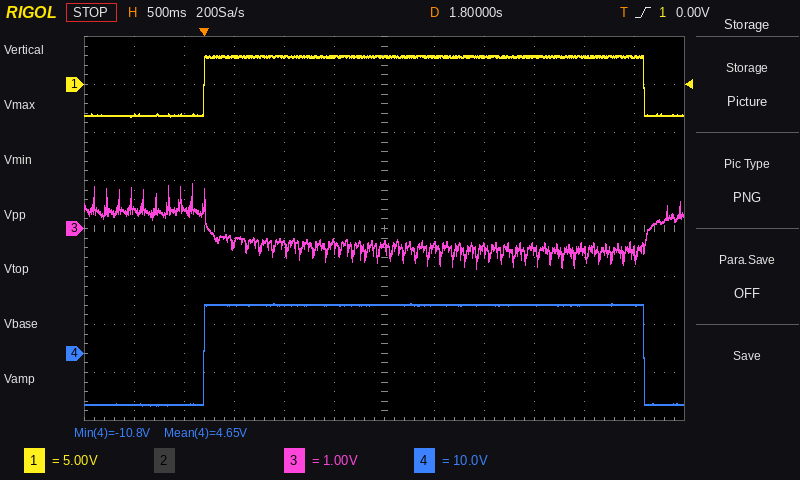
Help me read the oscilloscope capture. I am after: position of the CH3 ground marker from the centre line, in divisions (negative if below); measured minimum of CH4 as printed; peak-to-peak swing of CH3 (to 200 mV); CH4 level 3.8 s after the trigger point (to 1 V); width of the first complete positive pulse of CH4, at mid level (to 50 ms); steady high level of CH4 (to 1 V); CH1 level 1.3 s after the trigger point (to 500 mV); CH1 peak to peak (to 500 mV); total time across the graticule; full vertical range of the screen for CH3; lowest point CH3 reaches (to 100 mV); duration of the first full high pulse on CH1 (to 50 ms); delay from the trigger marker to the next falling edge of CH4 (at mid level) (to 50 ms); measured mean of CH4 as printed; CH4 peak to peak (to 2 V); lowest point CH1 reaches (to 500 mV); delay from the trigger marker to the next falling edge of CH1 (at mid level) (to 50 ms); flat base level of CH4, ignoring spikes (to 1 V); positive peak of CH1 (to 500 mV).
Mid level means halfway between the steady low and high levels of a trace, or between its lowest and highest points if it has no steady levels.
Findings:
0.0 div
-10.8 V
1.8 V
10 V
4.40 s
10 V
3.0 V
6.5 V
6 s
8 V
-800 mV
4.40 s
4.40 s
4.65 V
22 V
-3.5 V
4.40 s
-11 V
3.0 V
